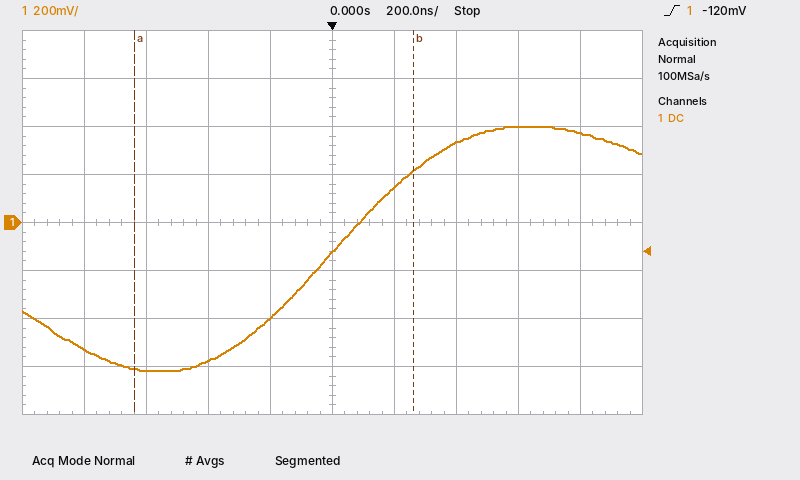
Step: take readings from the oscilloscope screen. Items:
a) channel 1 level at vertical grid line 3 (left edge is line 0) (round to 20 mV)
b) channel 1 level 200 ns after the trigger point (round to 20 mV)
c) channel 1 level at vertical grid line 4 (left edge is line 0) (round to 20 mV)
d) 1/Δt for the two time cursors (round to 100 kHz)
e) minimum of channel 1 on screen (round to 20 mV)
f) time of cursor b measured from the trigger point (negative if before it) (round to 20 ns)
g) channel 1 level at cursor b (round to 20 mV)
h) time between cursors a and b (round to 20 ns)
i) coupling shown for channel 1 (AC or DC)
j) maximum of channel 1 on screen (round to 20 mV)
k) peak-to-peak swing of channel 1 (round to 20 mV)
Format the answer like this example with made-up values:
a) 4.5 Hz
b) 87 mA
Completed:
a) -580 mV
b) 140 mV
c) -400 mV
d) 1.1 MHz
e) -620 mV
f) +260 ns
g) 220 mV
h) 900 ns
i) DC
j) 400 mV
k) 1.02 V
